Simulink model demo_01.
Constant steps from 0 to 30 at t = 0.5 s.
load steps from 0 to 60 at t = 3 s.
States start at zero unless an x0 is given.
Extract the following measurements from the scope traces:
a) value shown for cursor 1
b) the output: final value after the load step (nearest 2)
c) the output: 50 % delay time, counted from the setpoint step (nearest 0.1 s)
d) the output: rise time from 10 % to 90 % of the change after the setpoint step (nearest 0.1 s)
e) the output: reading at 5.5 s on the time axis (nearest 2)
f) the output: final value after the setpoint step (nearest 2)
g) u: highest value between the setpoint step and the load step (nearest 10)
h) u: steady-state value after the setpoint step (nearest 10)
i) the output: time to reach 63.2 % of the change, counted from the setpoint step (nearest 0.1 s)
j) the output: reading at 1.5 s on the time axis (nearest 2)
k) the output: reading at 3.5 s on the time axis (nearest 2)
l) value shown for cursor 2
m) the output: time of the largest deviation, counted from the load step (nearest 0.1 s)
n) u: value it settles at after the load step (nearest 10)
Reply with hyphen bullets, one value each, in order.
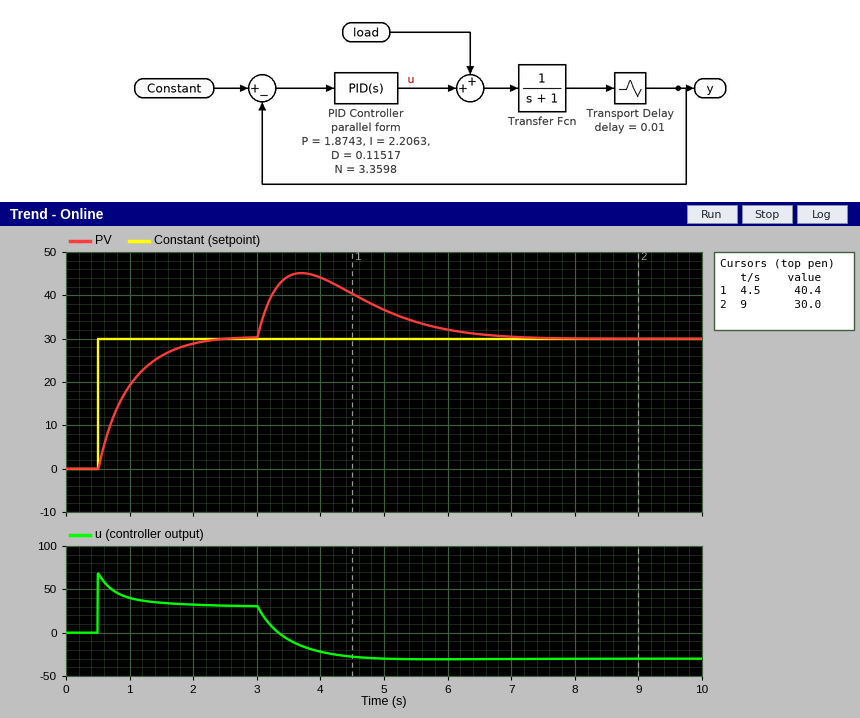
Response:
- 40.4
- 30
- 0.3 s
- 1.1 s
- 34
- 30
- 70
- 30
- 0.5 s
- 26
- 44
- 30.0
- 0.7 s
- -30
